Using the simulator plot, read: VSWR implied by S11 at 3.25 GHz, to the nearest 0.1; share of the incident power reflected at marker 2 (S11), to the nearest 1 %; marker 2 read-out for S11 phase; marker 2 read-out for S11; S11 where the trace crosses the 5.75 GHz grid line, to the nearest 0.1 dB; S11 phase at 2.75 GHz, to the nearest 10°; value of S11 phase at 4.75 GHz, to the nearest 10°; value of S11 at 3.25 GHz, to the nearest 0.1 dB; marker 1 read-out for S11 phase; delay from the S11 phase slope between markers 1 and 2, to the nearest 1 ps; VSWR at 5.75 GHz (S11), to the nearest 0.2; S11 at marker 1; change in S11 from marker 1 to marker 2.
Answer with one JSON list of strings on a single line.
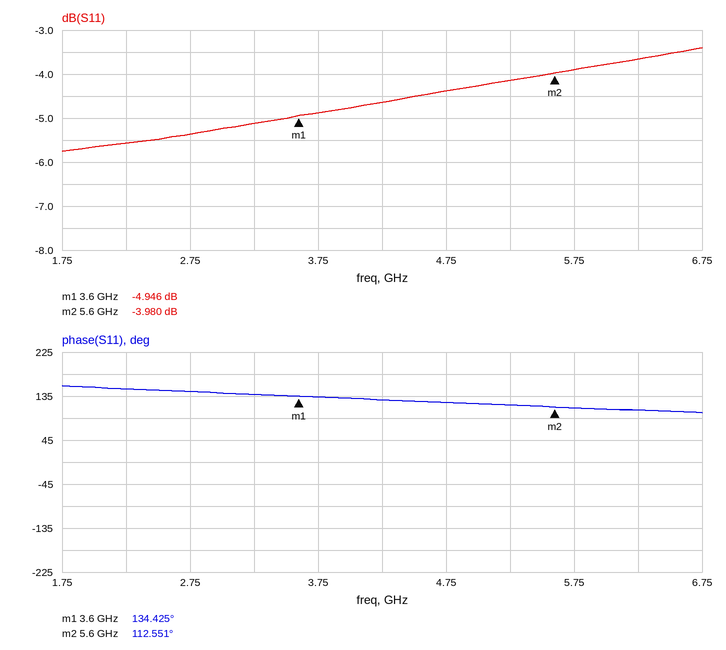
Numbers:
["3.5", "40 %", "112.551°", "-3.980 dB", "-3.9 dB", "140°", "120°", "-5.1 dB", "134.425°", "30 ps", "4.6", "-4.946 dB", "0.966 dB"]
